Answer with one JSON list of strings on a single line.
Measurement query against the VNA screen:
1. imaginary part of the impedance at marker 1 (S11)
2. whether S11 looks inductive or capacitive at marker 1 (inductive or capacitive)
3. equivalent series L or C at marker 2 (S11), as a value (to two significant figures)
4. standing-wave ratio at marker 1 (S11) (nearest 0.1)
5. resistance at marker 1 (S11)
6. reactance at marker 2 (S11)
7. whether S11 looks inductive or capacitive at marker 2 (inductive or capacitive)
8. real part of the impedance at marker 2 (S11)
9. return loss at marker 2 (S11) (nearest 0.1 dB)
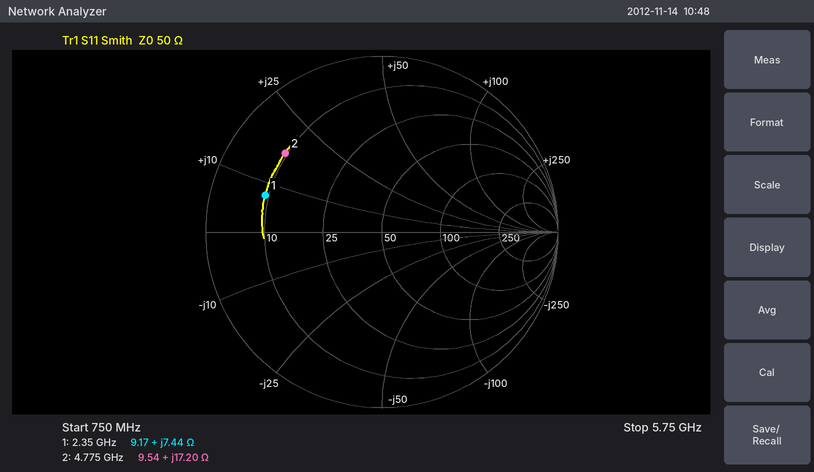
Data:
["+7.44 Ω", "inductive", "570 pH", "5.6", "9.17 Ω", "+17.20 Ω", "inductive", "9.54 Ω", "3.0 dB"]
